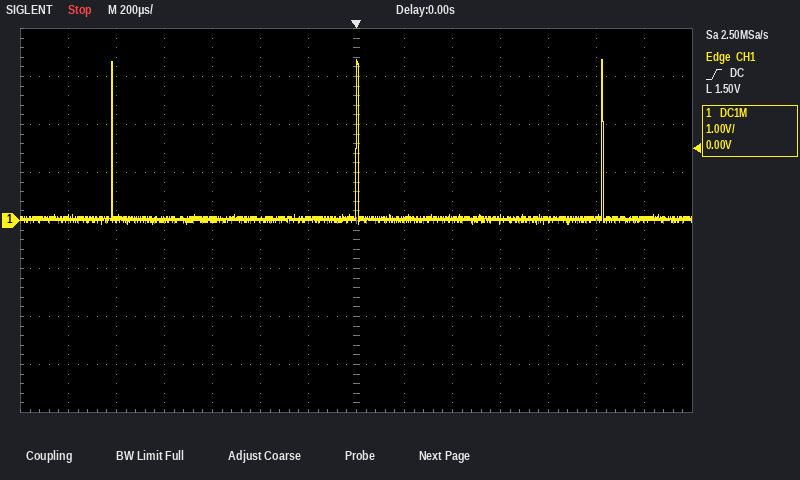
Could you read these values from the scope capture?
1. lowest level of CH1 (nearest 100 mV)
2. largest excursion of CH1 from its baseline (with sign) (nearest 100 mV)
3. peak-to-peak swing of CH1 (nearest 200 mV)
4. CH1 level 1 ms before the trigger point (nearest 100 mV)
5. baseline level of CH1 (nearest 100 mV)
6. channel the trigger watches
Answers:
-100 mV
+3.3 V
3.4 V
0.0 V
0.0 V
CH1
